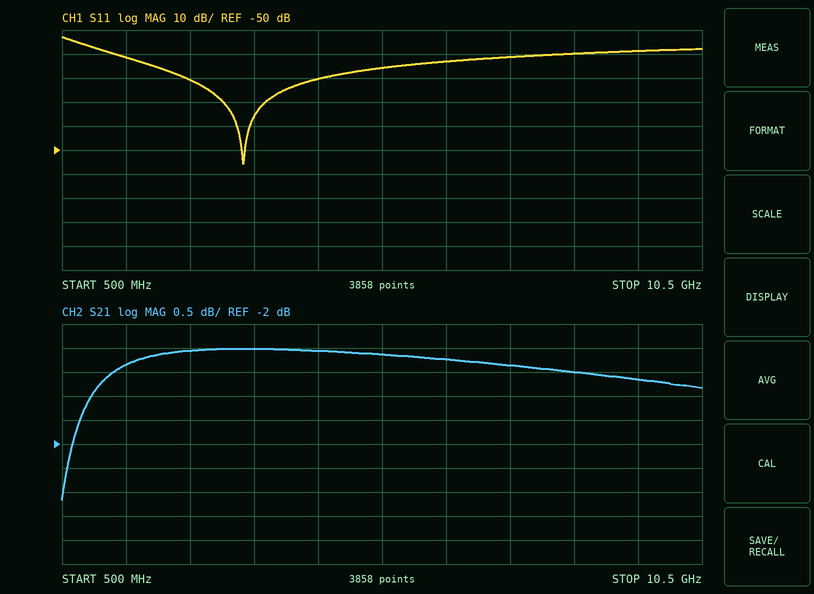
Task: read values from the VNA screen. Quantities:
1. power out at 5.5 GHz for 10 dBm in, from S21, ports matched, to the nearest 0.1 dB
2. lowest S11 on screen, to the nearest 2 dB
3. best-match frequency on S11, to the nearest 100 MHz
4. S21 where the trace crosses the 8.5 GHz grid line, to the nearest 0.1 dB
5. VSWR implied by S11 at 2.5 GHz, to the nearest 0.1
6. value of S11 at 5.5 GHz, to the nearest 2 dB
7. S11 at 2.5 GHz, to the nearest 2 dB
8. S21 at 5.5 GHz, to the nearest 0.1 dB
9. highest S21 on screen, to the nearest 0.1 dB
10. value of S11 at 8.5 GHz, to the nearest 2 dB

9.9 dBm
-56 dB
3.3 GHz
-0.5 dB
1.2
-16 dB
-20 dB
-0.1 dB
0.0 dB
-10 dB
